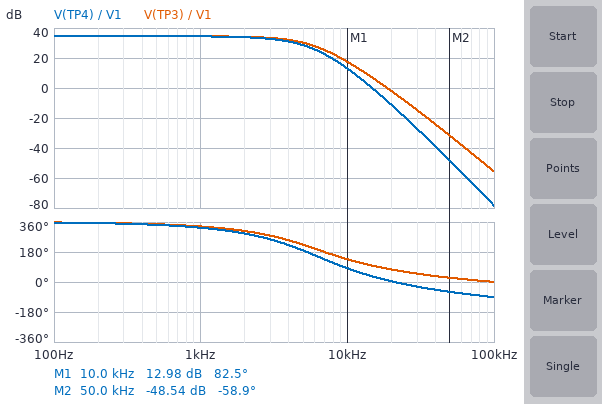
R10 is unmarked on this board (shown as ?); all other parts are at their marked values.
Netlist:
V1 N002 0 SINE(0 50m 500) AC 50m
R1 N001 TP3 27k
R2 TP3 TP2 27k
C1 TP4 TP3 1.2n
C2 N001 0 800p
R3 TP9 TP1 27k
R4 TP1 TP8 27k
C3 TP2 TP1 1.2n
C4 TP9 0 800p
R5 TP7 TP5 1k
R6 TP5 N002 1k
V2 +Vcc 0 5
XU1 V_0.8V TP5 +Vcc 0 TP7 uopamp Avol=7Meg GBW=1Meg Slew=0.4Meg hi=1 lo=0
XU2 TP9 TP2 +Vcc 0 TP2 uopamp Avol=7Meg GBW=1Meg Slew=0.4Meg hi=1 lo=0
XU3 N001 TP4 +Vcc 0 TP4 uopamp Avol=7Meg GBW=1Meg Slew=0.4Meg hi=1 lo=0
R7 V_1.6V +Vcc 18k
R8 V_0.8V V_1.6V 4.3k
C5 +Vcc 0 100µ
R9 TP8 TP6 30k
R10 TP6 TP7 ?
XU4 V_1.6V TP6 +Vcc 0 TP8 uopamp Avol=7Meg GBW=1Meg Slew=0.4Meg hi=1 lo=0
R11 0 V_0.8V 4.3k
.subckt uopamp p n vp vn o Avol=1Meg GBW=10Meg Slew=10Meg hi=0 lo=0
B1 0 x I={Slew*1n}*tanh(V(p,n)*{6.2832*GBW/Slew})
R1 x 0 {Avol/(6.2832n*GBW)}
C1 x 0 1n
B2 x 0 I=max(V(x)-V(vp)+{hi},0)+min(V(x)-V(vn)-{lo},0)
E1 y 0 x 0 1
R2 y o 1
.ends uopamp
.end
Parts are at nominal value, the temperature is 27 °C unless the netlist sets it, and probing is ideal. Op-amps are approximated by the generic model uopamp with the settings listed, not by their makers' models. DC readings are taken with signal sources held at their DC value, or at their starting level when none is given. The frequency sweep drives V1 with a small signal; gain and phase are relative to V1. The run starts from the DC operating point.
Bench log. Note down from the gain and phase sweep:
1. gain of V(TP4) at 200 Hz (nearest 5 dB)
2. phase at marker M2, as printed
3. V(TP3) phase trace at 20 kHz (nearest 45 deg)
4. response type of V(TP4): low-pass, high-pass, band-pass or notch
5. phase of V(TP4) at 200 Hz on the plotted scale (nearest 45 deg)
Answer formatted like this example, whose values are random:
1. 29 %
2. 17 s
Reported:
1. 35 dB
2. -58.9 deg
3. 90 deg
4. low-pass
5. 360 deg
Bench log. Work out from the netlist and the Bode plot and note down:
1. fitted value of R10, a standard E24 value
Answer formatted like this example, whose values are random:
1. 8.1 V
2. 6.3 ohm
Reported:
1. 560 Ω
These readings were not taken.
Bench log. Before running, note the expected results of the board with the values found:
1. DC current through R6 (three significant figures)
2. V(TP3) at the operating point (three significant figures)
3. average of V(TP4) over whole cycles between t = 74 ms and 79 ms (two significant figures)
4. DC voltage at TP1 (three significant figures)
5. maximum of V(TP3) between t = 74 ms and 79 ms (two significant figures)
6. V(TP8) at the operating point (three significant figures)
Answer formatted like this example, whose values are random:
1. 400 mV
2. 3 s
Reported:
1. 808 µA
2. 1.62 V
3. 1.8 V
4. 1.62 V
5. 4.0 V
6. 1.62 V
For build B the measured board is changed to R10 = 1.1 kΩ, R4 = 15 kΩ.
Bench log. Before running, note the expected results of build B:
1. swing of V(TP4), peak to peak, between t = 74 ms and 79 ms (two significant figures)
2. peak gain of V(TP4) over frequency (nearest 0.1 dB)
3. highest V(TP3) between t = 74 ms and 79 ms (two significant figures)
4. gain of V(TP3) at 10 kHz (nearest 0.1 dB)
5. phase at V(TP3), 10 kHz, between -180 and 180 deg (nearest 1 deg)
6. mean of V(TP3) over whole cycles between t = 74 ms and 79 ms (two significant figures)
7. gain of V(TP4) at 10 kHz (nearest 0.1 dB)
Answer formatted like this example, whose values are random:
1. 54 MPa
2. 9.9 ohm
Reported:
1. 2.7 V
2. 28.7 dB
3. 3.0 V
4. 15.9 dB
5. 168 deg
6. 1.6 V
7. 11.4 dB
